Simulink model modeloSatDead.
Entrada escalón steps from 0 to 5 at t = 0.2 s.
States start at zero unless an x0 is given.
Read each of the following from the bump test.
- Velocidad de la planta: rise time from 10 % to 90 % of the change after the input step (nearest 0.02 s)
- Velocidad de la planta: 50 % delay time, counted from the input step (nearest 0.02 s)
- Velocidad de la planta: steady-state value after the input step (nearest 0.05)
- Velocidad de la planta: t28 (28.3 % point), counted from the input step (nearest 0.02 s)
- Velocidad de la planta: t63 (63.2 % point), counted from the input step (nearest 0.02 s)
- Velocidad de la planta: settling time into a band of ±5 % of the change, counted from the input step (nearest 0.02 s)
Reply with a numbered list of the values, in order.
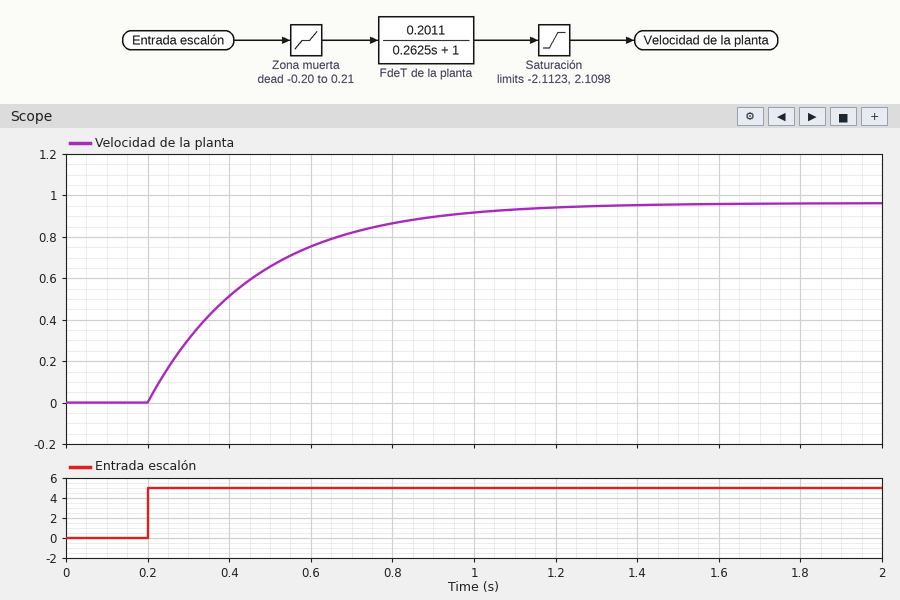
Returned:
1. 0.58 s
2. 0.18 s
3. 0.95
4. 0.08 s
5. 0.26 s
6. 0.78 s
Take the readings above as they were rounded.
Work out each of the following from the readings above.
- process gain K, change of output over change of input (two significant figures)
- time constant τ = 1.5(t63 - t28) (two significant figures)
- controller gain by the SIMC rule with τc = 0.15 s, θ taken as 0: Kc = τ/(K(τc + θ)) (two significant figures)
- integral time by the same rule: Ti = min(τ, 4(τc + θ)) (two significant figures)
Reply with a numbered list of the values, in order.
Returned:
1. 0.19
2. 0.27 s
3. 9.5
4. 0.27 s
